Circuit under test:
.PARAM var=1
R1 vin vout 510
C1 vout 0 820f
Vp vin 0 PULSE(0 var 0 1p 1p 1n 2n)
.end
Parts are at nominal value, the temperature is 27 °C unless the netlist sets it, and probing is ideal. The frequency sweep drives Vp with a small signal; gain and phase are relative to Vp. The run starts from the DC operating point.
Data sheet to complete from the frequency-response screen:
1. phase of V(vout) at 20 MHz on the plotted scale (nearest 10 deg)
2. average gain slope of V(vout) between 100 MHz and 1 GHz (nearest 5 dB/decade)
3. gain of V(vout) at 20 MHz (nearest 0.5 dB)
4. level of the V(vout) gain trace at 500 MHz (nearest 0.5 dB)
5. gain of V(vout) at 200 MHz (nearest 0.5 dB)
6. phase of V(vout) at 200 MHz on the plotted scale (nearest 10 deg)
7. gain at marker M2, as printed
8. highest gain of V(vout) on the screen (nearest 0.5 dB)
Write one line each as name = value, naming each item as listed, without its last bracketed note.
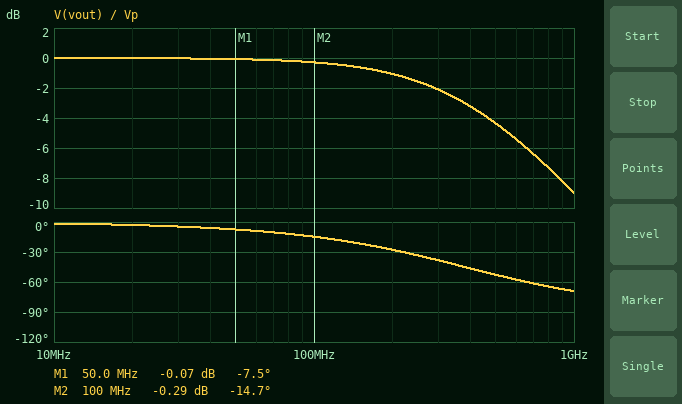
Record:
phase of V(vout) at 20 MHz on the plotted scale = 0 deg
average gain slope of V(vout) between 100 MHz and 1 GHz = -10 dB/decade
gain of V(vout) at 20 MHz = 0 dB
level of the V(vout) gain trace at 500 MHz = -4.5 dB
gain of V(vout) at 200 MHz = -1.0 dB
phase of V(vout) at 200 MHz on the plotted scale = -30 deg
gain at marker M2, as printed = -0.29 dB
highest gain of V(vout) on the screen = 0 dB
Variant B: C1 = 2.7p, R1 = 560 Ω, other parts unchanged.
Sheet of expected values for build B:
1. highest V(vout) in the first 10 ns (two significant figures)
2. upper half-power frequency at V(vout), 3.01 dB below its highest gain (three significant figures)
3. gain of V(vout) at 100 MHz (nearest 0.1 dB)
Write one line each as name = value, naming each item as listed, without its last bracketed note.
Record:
highest V(vout) in the first 10 ns = 660 mV
upper half-power frequency at V(vout), 3.01 dB below its highest gain = 105 MHz
gain of V(vout) at 100 MHz = -2.8 dB
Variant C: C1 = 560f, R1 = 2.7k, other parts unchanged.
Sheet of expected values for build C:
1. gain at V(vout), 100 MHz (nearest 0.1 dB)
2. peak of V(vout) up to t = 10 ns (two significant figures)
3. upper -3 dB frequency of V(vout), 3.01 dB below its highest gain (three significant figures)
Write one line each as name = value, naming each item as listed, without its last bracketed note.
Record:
gain at V(vout), 100 MHz = -2.8 dB
peak of V(vout) up to t = 10 ns = 660 mV
upper -3 dB frequency of V(vout), 3.01 dB below its highest gain = 105 MHz
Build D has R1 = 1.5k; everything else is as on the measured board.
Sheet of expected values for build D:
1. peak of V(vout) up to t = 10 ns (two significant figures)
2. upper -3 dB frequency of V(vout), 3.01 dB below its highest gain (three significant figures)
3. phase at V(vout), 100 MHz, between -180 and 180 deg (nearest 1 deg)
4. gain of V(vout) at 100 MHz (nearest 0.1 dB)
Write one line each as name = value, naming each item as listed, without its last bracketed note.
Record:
peak of V(vout) up to t = 10 ns = 690 mV
upper -3 dB frequency of V(vout), 3.01 dB below its highest gain = 129 MHz
phase at V(vout), 100 MHz, between -180 and 180 deg = -38 deg
gain of V(vout) at 100 MHz = -2.0 dB
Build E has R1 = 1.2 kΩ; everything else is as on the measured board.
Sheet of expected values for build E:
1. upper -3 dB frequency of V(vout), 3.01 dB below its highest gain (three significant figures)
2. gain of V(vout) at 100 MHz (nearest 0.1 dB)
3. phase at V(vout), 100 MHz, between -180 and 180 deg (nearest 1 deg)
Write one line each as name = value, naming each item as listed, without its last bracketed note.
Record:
upper -3 dB frequency of V(vout), 3.01 dB below its highest gain = 162 MHz
gain of V(vout) at 100 MHz = -1.4 dB
phase at V(vout), 100 MHz, between -180 and 180 deg = -32 deg
